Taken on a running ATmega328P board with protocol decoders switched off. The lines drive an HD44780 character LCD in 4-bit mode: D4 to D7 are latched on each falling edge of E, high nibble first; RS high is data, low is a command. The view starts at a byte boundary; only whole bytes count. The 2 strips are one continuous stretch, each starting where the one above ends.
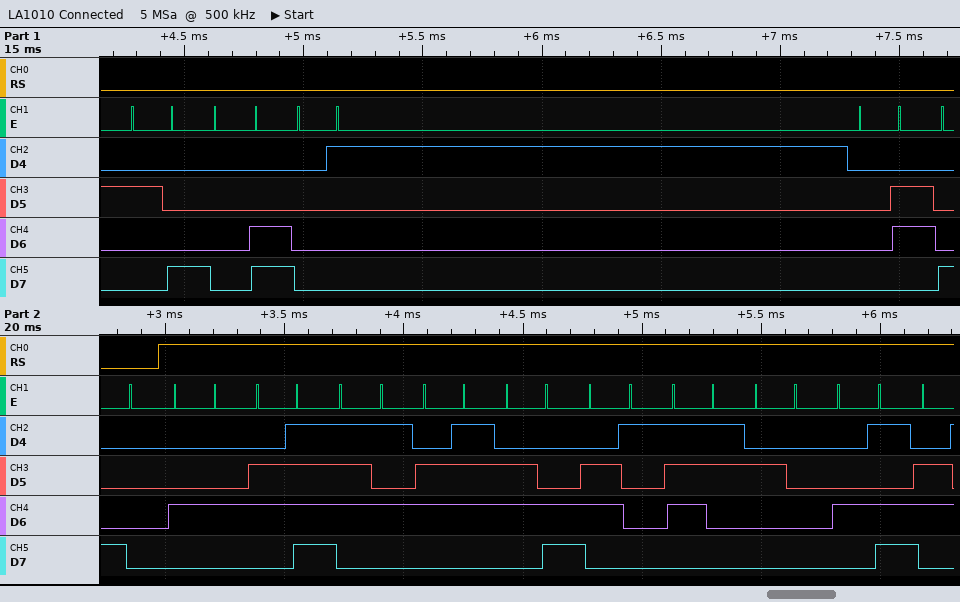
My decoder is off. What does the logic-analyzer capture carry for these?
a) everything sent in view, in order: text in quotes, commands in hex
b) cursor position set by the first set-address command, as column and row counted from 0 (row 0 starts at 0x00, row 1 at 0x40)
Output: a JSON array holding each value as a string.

["0x28 0x0C 0x01 0x06 0x80 \"Douglas M\"", "column 0, row 0"]
